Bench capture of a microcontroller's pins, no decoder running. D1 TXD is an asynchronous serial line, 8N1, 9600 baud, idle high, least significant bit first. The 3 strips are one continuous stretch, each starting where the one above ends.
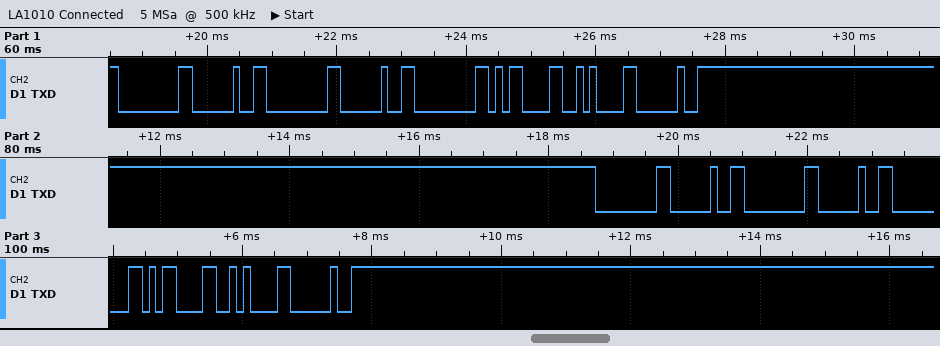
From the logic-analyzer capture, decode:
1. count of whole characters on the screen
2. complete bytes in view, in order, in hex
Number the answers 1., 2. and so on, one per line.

1. 16
2. 0x00 0x20 0x00 0x20 0x00 0x0D 0x0A 0x20 0x00 0x20 0x00 0x20 0x00 0x0D 0x0A 0x20
